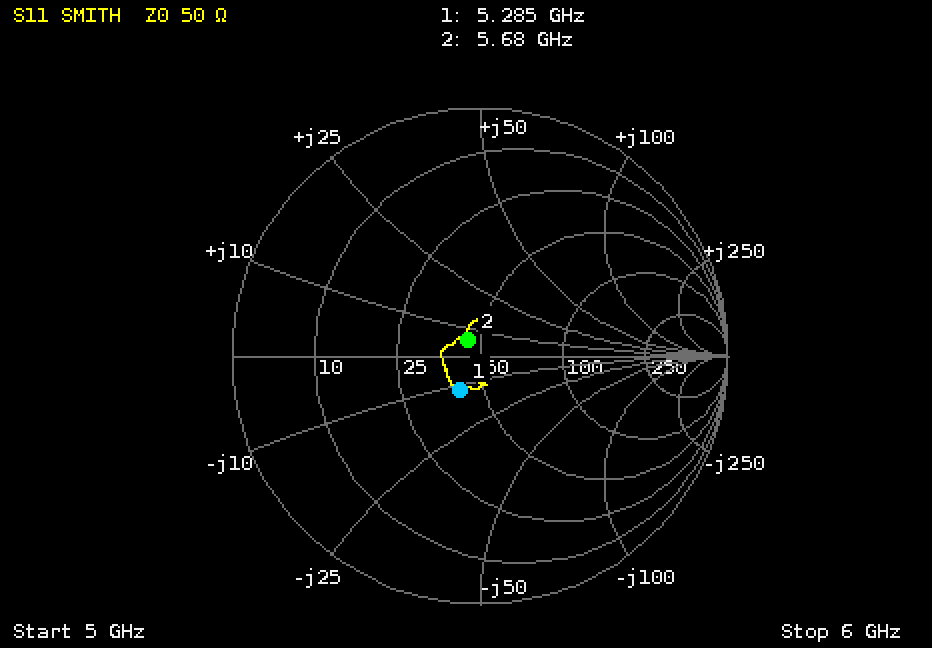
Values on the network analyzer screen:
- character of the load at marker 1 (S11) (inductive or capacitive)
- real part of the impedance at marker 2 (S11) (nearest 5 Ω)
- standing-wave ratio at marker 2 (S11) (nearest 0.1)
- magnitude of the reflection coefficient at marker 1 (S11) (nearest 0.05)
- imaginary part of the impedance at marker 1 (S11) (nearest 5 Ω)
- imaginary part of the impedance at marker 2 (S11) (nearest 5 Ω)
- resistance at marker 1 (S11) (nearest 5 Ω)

capacitive
45 Ω
1.2
0.15
-10 Ω
+5 Ω
40 Ω
